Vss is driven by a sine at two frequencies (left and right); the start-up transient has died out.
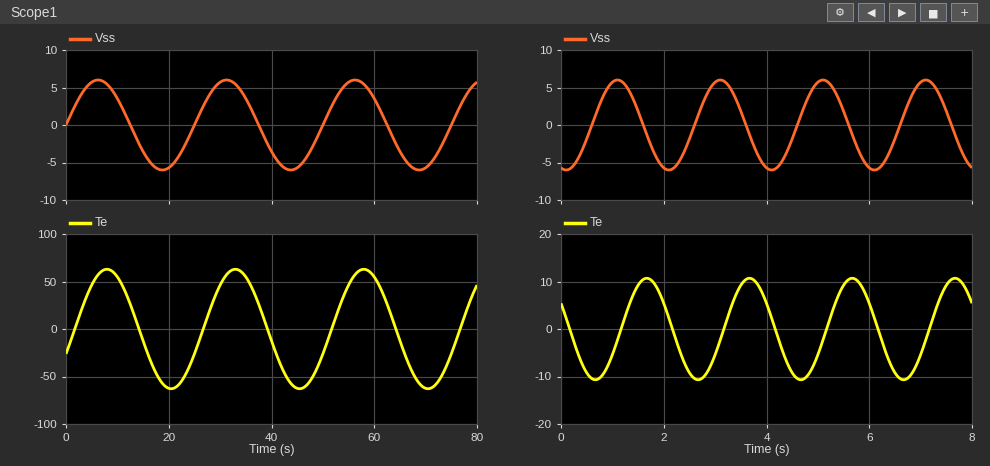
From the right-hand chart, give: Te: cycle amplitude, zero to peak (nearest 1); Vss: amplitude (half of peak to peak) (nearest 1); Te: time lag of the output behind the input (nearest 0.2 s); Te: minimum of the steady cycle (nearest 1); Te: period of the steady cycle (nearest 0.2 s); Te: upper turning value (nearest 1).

11
6
0.6 s
-11
2.0 s
11
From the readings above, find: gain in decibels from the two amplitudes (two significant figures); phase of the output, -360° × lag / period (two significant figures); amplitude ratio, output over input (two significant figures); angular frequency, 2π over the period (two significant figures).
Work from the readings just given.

5.3 dB
-110°
1.8
3.1 rad/s
